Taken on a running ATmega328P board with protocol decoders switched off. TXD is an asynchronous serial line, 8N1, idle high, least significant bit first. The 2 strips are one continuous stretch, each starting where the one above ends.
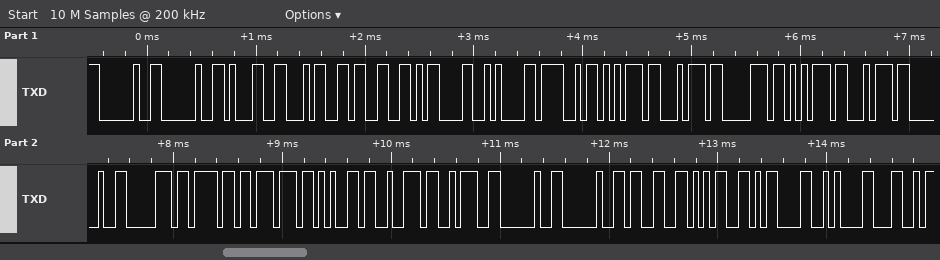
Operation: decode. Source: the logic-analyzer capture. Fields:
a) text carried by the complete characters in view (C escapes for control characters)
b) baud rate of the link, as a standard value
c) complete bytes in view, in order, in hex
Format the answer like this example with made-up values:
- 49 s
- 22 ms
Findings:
- "  143\r\nOutput power:  35\r\nL"
- 19200 baud
- 20 20 31 34 33 0D 0A 4F 75 74 70 75 74 20 70 6F 77 65 72 3A 20 20 33 35 0D 0A 4C
